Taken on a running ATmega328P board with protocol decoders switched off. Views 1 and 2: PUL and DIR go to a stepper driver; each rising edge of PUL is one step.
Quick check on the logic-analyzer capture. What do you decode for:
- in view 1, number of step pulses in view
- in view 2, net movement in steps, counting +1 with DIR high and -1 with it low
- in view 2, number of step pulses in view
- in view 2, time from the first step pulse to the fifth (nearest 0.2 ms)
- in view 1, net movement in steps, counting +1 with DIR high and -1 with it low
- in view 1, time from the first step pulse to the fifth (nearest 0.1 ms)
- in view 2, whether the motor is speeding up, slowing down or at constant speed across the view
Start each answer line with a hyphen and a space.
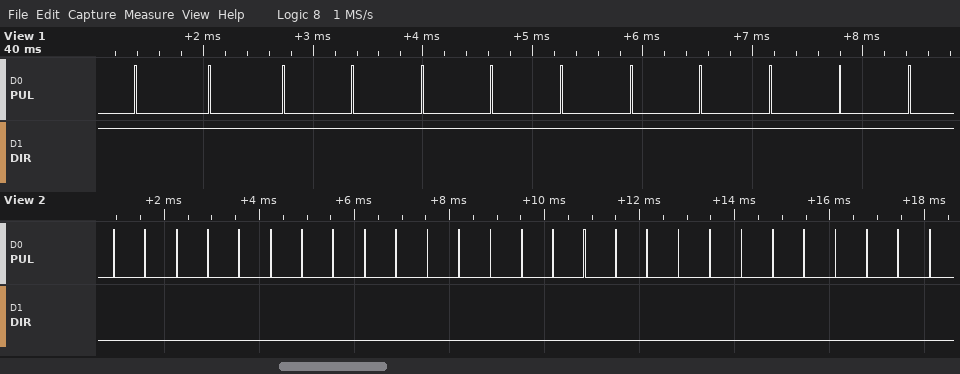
- 12
- -27
- 27
- 2.6 ms
- +12
- 2.6 ms
- constant speed
